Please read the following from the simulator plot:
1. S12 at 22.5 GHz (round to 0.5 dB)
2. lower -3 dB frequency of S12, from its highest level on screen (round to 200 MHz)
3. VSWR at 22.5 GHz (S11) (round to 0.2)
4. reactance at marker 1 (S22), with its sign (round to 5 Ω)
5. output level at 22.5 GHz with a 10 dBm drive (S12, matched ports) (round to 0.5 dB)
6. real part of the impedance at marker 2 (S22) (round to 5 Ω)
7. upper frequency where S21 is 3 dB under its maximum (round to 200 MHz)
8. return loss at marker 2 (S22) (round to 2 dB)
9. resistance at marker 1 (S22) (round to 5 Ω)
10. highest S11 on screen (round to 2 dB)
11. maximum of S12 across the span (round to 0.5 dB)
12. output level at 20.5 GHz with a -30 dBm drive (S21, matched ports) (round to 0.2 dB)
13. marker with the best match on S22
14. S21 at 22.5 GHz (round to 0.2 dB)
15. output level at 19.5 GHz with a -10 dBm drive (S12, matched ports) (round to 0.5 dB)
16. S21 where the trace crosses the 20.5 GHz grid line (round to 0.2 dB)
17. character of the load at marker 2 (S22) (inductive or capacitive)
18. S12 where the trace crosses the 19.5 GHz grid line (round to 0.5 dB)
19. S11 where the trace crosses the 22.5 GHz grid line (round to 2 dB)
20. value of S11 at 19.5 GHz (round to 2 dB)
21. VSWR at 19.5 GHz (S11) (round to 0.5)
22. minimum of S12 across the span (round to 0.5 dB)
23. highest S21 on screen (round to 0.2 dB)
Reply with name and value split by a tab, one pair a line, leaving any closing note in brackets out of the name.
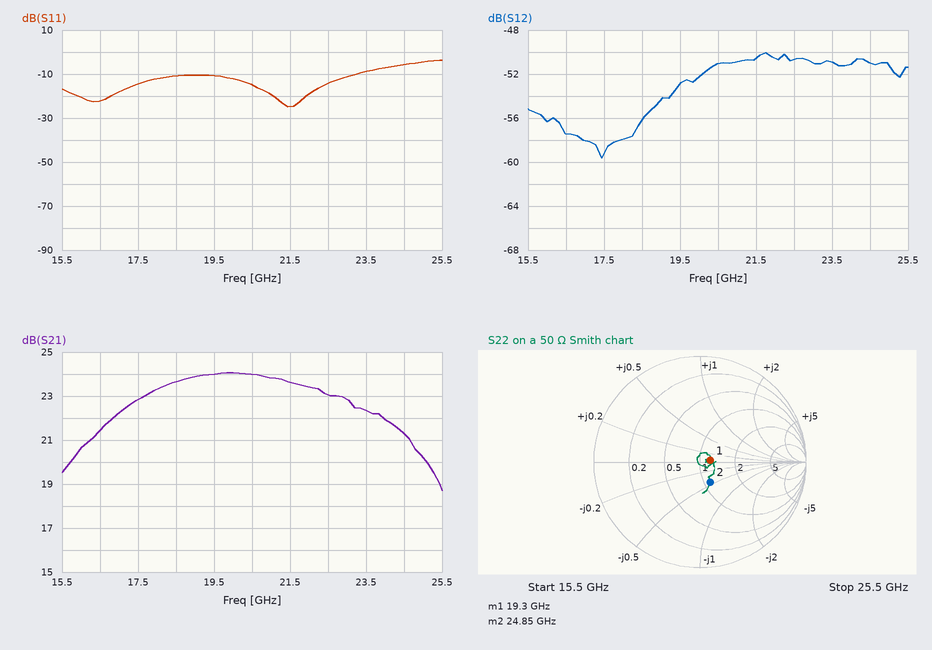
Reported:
S12 at 22.5 GHz	-50.5 dB
lower -3 dB frequency of S12, from its highest level on screen	19.4 GHz
VSWR at 22.5 GHz (S11)	1.4
reactance at marker 1 (S22), with its sign	0 Ω
output level at 22.5 GHz with a 10 dBm drive (S12, matched ports)	-40.5 dBm
real part of the impedance at marker 2 (S22)	55 Ω
upper frequency where S21 is 3 dB under its maximum	24.6 GHz
return loss at marker 2 (S22)	14 dB
resistance at marker 1 (S22)	60 Ω
highest S11 on screen	-4 dB
maximum of S12 across the span	-50.0 dB
output level at 20.5 GHz with a -30 dBm drive (S21, matched ports)	-6.0 dBm
marker with the best match on S22	marker 1
S21 at 22.5 GHz	23.0 dB
output level at 19.5 GHz with a -10 dBm drive (S12, matched ports)	-63.0 dBm
S21 where the trace crosses the 20.5 GHz grid line	24.0 dB
character of the load at marker 2 (S22)	capacitive
S12 where the trace crosses the 19.5 GHz grid line	-53.0 dB
S11 where the trace crosses the 22.5 GHz grid line	-14 dB
value of S11 at 19.5 GHz	-10 dB
VSWR at 19.5 GHz (S11)	2.0
minimum of S12 across the span	-59.5 dB
highest S21 on screen	24.0 dB
